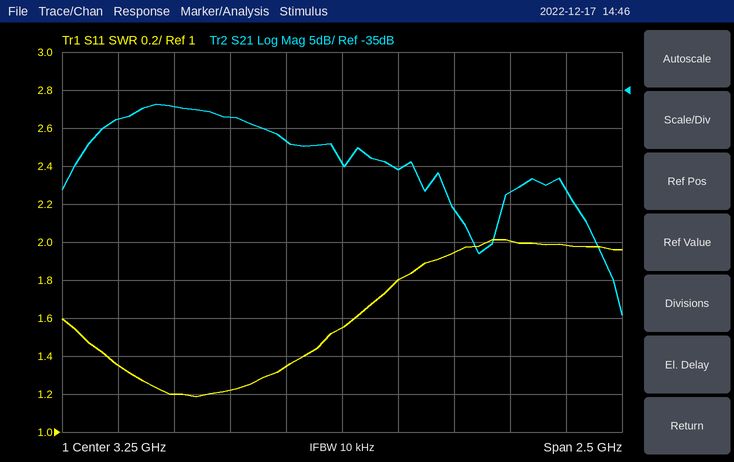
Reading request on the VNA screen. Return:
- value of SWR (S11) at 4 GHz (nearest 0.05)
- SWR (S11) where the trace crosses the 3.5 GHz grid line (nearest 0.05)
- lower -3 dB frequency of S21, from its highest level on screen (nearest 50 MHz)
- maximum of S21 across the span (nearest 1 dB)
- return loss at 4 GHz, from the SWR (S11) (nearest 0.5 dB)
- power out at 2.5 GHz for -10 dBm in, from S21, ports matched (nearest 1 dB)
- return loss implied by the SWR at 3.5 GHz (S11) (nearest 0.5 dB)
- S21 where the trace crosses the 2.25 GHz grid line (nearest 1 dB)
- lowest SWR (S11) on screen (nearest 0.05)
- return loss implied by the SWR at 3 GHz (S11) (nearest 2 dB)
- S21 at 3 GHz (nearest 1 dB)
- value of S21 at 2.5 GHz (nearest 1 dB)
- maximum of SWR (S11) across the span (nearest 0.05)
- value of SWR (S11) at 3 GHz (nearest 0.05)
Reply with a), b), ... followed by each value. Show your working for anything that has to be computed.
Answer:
a) 2.00
b) 1.80
c) 2.20 GHz
d) -37 dB
e) −20 log10((2 − 1)/(2 + 1)) ≈ 9.5 dB
f) -10 dBm + (-37 dB) = -47 dBm
g) −20 log10((1.8 − 1)/(1.8 + 1)) ≈ 10.9 dB, so 11.0 dB to the nearest 0.5 dB
h) -39 dB
i) 1.20
j) −20 log10((1.35 − 1)/(1.35 + 1)) ≈ 16 dB
k) -42 dB
l) -37 dB
m) 2.00
n) 1.35
